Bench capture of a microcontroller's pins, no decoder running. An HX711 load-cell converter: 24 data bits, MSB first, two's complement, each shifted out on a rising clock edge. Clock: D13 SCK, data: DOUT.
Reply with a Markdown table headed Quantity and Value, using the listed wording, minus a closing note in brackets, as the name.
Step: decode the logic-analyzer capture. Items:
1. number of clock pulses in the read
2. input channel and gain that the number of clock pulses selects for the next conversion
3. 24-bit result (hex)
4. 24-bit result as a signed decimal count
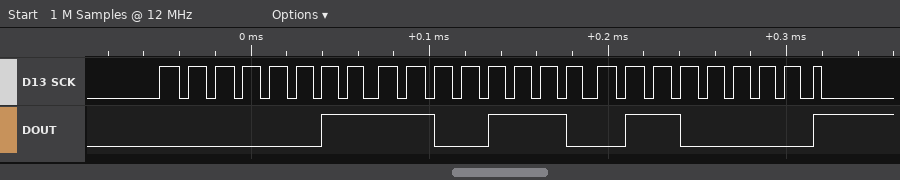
| Quantity | Value |
|---|---|
| number of clock pulses in the read | 25 |
| input channel and gain that the number of clock pulses selects for the next conversion | channel A, gain 128 |
| 24-bit result | 0x03CE60 |
| 24-bit result as a signed decimal count | 249440 |
